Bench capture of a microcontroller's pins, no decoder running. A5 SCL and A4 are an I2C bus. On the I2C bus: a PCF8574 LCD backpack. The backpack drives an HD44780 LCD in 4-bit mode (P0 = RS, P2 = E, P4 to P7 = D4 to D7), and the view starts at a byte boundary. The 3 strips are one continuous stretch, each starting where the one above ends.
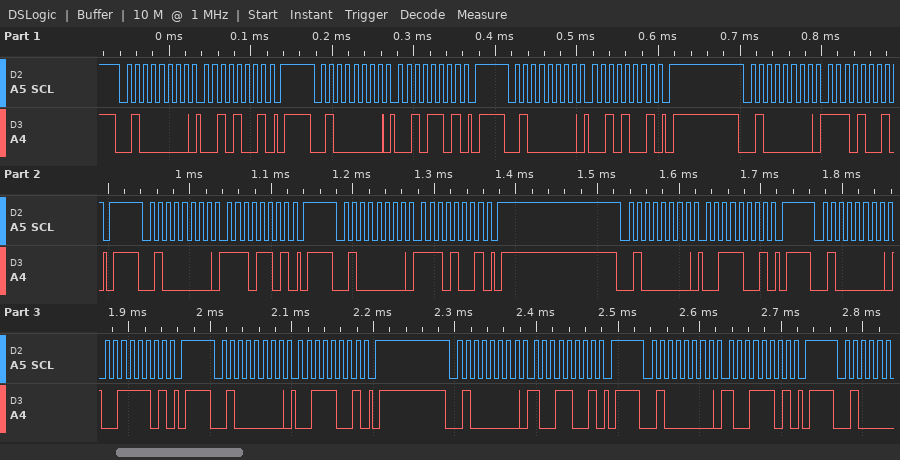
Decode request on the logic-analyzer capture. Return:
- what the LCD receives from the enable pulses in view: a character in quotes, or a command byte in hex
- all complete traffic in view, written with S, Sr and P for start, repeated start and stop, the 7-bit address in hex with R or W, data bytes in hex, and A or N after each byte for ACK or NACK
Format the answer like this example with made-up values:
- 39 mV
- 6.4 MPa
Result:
- '.'
- S 20W A 29 A P S 20W A 2D A P S 20W A 29 A P S 20W A E9 A P S 20W A ED A P S 20W A E9 A P S 20W A 39 A P S 20W A 3D A P S 20W A 39 A P S 20W A 99 A P S 20W A 9D A P
